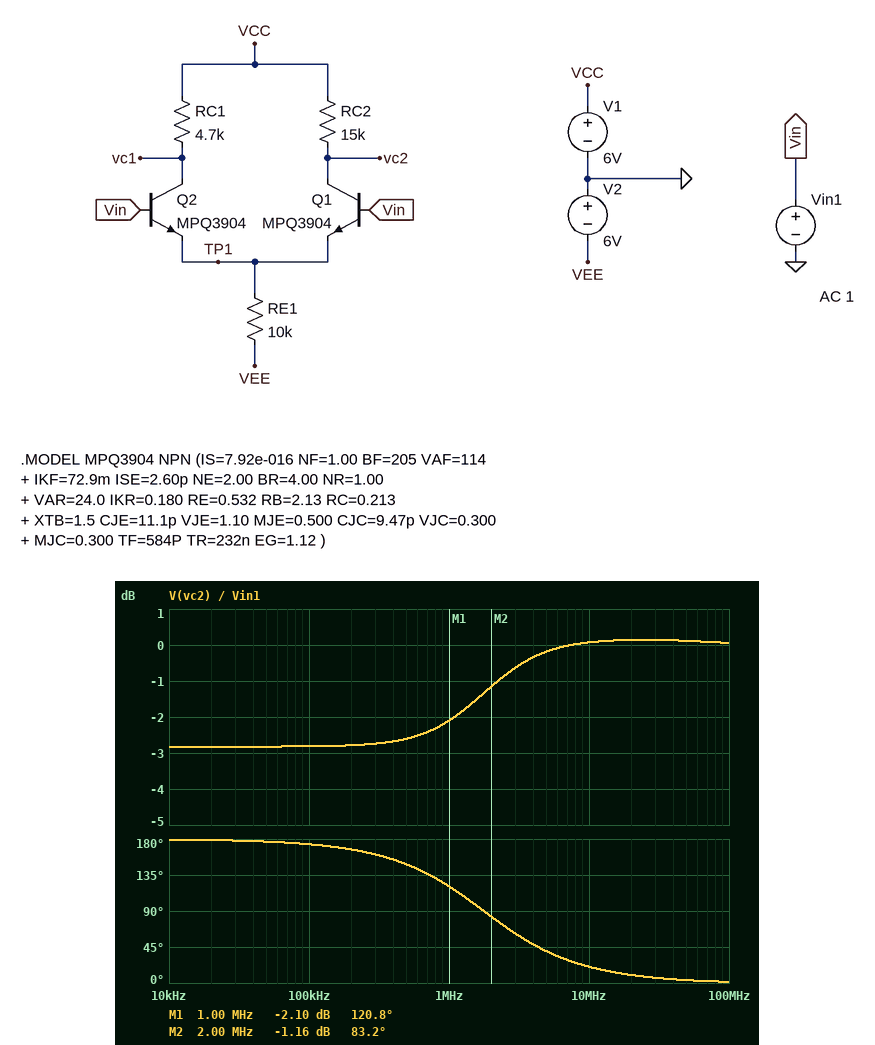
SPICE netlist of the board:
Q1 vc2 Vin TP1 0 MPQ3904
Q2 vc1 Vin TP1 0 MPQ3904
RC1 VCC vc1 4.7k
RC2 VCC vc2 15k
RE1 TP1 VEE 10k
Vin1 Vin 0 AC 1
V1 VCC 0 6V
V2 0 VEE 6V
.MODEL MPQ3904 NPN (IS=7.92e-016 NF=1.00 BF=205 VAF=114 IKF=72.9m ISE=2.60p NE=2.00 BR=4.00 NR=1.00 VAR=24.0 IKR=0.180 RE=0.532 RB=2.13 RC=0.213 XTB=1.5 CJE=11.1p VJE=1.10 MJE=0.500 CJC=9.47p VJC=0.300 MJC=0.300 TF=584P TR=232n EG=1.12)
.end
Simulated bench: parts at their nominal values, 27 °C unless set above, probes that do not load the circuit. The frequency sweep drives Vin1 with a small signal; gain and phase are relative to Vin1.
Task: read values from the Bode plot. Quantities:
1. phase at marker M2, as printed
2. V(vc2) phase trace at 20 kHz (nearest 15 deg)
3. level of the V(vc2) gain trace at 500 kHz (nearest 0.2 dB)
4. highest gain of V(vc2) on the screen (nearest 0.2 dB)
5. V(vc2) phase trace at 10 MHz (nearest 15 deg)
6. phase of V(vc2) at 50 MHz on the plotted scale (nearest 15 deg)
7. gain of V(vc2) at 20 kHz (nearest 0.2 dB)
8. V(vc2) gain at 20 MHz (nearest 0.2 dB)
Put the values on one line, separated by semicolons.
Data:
83.2 deg; 180 deg; -2.6 dB; 0.2 dB; 15 deg; 0 deg; -2.8 dB; 0.2 dB
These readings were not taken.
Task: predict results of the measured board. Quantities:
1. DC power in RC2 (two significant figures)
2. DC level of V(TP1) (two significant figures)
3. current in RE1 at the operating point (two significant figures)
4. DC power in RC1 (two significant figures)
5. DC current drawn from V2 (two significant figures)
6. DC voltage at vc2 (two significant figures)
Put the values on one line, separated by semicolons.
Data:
1.0 mW; -690 mV; 530 µA; 330 µW; 530 µA; 2.1 V
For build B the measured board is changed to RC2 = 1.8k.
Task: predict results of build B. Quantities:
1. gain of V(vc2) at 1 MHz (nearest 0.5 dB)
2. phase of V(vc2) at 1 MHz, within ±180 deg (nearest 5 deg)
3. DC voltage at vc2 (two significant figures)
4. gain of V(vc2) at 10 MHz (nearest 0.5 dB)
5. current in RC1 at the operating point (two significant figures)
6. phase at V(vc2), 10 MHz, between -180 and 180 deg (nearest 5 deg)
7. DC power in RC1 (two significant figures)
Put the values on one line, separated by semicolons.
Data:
-20.0 dB; 150 deg; 5.5 V; -7.5 dB; 260 µA; 75 deg; 320 µW
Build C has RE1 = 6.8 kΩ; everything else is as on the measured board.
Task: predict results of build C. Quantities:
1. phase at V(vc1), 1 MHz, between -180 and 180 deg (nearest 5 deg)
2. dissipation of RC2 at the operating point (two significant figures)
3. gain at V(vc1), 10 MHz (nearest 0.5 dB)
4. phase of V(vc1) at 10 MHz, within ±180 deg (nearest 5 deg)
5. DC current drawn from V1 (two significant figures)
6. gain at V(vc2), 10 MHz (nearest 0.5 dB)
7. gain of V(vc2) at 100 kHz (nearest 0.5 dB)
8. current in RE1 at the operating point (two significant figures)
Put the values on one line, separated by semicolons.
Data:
150 deg; 2.2 mW; -1.5 dB; 55 deg; 770 µA; 0 dB; 0.5 dB; 780 µA
